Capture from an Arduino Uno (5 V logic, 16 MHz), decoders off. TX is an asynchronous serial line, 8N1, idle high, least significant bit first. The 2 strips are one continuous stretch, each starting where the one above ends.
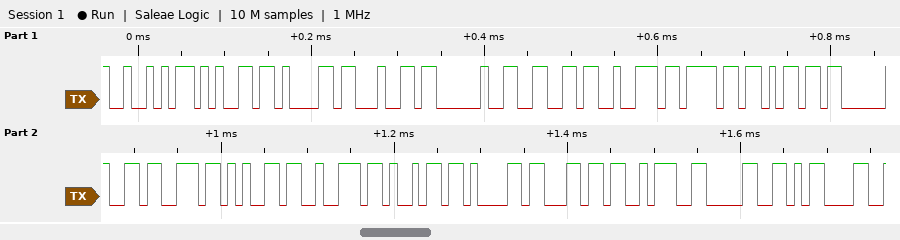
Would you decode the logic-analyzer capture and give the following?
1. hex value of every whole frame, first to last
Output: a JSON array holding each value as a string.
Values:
["0x52 0x65 0x61 0x64 0x20 0x66 0x72 0x6F 0x6D 0x20 0x73 0x65 0x72 0x69 0x61 0x6C 0x3A 0x30 0x0D"]
